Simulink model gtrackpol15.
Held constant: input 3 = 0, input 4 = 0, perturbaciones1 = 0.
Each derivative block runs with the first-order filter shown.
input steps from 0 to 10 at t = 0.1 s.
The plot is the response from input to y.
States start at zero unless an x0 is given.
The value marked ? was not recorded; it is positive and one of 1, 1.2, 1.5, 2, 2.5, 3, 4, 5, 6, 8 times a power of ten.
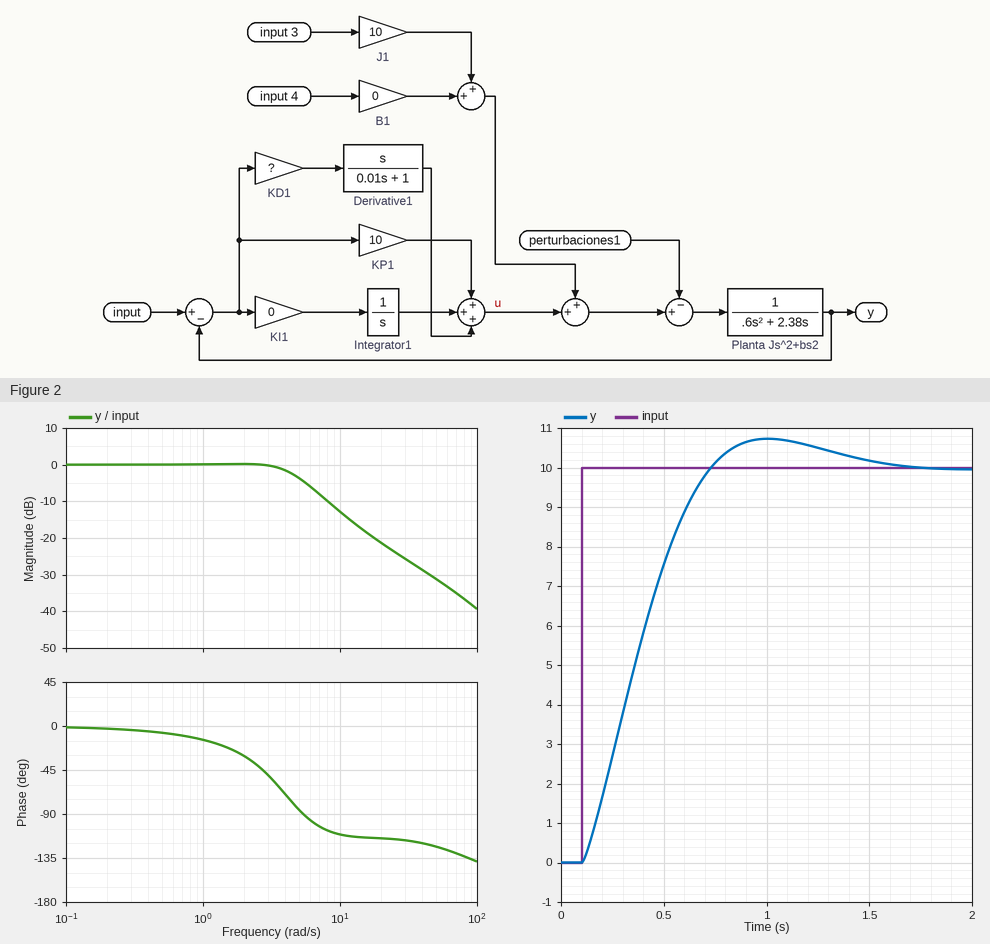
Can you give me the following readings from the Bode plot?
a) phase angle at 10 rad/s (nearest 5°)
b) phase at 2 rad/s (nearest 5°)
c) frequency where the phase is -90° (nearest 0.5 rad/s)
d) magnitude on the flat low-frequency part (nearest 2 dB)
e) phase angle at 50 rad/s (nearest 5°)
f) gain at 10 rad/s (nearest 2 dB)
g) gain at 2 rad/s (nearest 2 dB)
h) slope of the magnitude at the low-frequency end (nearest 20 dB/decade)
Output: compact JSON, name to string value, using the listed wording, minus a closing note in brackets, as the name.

{"phase angle at 10 rad/s": "-110°", "phase at 2 rad/s": "-30°", "frequency where the phase is -90°": "5.5 rad/s", "magnitude on the flat low-frequency part": "0 dB", "phase angle at 50 rad/s": "-125°", "gain at 10 rad/s": "-12 dB", "gain at 2 rad/s": "0 dB", "slope of the magnitude at the low-frequency end": "0 dB/decade"}
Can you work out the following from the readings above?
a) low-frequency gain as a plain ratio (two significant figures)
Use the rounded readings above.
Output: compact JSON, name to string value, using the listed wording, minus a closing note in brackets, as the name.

{"low-frequency gain as a plain ratio": "1.0"}
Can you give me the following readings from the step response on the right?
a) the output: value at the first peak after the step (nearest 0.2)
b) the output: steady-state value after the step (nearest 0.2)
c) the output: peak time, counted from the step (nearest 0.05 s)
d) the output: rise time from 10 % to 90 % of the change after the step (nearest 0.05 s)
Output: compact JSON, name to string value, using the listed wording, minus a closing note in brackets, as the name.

{"the output: value at the first peak after the step": "10.8", "the output: steady-state value after the step": "10.0", "the output: peak time, counted from the step": "0.90 s", "the output: rise time from 10 % to 90 % of the change after the step": "0.45 s"}
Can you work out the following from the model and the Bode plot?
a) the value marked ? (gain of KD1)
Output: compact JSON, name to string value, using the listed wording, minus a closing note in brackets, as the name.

{"the value marked ?": "0.8"}
